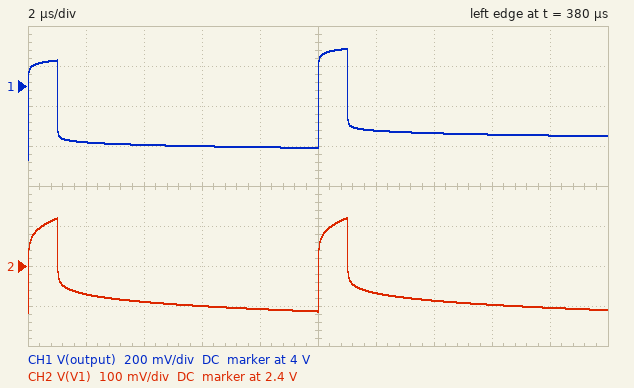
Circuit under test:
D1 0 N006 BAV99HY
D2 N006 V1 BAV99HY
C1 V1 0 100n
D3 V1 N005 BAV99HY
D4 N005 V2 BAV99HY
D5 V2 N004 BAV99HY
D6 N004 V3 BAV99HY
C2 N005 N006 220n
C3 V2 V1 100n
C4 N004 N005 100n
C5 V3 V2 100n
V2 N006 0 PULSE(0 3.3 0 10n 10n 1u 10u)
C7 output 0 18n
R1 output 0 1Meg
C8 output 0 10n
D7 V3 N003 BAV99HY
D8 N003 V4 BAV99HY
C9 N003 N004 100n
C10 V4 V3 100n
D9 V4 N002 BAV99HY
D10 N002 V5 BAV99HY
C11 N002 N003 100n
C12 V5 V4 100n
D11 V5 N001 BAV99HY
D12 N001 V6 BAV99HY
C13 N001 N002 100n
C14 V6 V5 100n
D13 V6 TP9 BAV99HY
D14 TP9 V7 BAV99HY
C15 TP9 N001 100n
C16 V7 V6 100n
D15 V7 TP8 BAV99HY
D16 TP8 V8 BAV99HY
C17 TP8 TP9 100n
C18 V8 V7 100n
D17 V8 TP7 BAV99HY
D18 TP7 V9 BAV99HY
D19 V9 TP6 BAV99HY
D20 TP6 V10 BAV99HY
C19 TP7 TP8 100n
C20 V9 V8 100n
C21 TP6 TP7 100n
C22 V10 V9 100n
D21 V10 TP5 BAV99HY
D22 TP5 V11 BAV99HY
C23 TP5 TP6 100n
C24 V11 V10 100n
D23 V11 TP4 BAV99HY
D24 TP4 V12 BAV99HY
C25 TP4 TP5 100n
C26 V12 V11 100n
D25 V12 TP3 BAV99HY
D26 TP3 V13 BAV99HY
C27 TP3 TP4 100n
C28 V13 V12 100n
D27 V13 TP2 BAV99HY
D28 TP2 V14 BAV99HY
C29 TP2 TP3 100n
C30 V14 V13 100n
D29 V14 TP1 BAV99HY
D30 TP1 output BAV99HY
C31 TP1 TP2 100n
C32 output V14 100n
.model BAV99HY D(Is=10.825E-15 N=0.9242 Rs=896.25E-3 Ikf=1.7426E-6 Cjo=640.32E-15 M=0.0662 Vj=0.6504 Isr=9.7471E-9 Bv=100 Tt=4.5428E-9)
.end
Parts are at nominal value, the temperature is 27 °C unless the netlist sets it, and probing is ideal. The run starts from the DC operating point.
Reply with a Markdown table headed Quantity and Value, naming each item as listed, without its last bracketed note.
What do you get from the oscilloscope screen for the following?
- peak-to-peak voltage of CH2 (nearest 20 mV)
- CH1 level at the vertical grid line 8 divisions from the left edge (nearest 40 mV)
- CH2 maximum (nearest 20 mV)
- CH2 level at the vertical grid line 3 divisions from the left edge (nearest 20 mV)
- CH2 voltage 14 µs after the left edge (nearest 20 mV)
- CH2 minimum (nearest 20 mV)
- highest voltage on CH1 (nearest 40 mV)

| Quantity | Value |
|---|---|
| peak-to-peak voltage of CH2 | 240 mV |
| CH1 level at the vertical grid line 8 divisions from the left edge | 3.76 V |
| CH2 maximum | 2.52 V |
| CH2 level at the vertical grid line 3 divisions from the left edge | 2.30 V |
| CH2 voltage 14 µs after the left edge | 2.32 V |
| CH2 minimum | 2.28 V |
| highest voltage on CH1 | 4.20 V |
